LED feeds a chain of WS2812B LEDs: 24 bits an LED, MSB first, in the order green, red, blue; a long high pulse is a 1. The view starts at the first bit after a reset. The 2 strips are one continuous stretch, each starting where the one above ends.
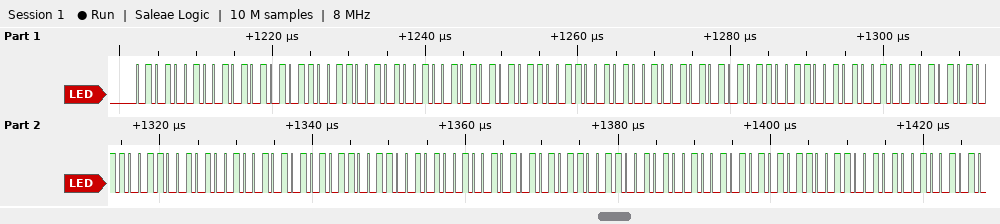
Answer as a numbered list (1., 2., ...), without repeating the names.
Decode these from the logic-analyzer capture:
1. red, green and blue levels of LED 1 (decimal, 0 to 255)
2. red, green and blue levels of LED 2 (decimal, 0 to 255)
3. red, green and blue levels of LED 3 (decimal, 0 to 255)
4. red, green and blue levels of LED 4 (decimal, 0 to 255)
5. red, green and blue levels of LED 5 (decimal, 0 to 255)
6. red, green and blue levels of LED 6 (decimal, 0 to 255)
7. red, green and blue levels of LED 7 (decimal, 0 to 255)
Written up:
1. 85, 82, 102
2. 85, 82, 102
3. 85, 82, 102
4. 85, 82, 102
5. 85, 82, 102
6. 85, 82, 102
7. 85, 82, 102
